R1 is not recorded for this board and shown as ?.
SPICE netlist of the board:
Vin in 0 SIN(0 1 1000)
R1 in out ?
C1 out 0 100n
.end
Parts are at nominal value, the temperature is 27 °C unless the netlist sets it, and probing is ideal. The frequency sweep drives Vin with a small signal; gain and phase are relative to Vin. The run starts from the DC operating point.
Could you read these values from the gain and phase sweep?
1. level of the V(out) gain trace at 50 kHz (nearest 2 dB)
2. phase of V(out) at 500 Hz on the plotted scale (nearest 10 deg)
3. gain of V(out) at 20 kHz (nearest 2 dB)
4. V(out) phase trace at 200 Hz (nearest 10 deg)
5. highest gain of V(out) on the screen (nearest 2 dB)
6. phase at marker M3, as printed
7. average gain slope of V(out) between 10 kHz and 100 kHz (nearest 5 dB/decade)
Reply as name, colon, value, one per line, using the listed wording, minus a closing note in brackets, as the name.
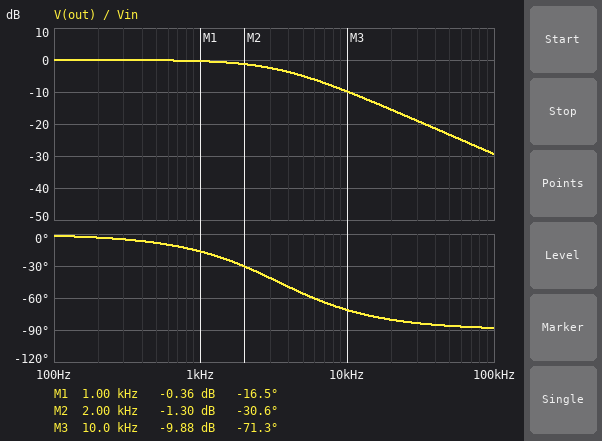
level of the V(out) gain trace at 50 kHz: -24 dB
phase of V(out) at 500 Hz on the plotted scale: -10 deg
gain of V(out) at 20 kHz: -16 dB
V(out) phase trace at 200 Hz: 0 deg
highest gain of V(out) on the screen: 0 dB
phase at marker M3, as printed: -71.3 deg
average gain slope of V(out) between 10 kHz and 100 kHz: -20 dB/decade
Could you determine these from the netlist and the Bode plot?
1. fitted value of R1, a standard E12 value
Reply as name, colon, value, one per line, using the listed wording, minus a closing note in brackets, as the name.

fitted value of R1, a standard E12 value: 470 Ω
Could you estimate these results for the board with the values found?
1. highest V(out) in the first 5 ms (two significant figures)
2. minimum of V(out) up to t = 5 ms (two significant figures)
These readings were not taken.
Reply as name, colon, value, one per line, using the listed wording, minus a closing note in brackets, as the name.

highest V(out) in the first 5 ms: 960 mV
minimum of V(out) up to t = 5 ms: -960 mV
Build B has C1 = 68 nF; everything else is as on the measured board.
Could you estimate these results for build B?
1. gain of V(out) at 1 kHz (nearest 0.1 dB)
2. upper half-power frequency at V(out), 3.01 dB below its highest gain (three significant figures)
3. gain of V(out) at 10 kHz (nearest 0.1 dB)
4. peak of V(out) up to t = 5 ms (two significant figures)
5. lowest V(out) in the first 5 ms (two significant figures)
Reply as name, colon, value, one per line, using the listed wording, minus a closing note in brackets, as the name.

gain of V(out) at 1 kHz: -0.2 dB
upper half-power frequency at V(out), 3.01 dB below its highest gain: 4.98 kHz
gain of V(out) at 10 kHz: -7.0 dB
peak of V(out) up to t = 5 ms: 980 mV
lowest V(out) in the first 5 ms: -980 mV
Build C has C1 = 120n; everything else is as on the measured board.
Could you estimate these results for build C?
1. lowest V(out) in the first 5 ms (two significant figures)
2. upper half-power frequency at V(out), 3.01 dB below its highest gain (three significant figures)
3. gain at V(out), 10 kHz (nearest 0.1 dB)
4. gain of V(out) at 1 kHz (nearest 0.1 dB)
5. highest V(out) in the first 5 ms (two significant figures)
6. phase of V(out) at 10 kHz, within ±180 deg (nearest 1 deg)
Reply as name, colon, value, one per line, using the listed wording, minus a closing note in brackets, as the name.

lowest V(out) in the first 5 ms: -940 mV
upper half-power frequency at V(out), 3.01 dB below its highest gain: 2.82 kHz
gain at V(out), 10 kHz: -11.3 dB
gain of V(out) at 1 kHz: -0.5 dB
highest V(out) in the first 5 ms: 940 mV
phase of V(out) at 10 kHz, within ±180 deg: -74 deg
